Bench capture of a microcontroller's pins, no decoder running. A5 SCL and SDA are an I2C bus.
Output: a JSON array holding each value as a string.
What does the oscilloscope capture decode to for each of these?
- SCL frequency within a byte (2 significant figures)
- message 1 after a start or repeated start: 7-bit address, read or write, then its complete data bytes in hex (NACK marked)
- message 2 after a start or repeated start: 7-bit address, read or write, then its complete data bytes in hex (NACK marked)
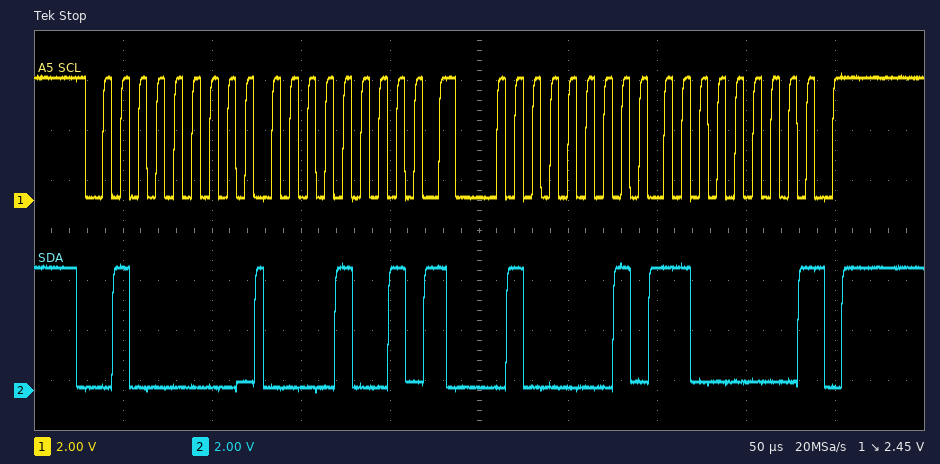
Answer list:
["100 kHz", "0x20 write: 09", "0x20 read: C0 NACK"]
